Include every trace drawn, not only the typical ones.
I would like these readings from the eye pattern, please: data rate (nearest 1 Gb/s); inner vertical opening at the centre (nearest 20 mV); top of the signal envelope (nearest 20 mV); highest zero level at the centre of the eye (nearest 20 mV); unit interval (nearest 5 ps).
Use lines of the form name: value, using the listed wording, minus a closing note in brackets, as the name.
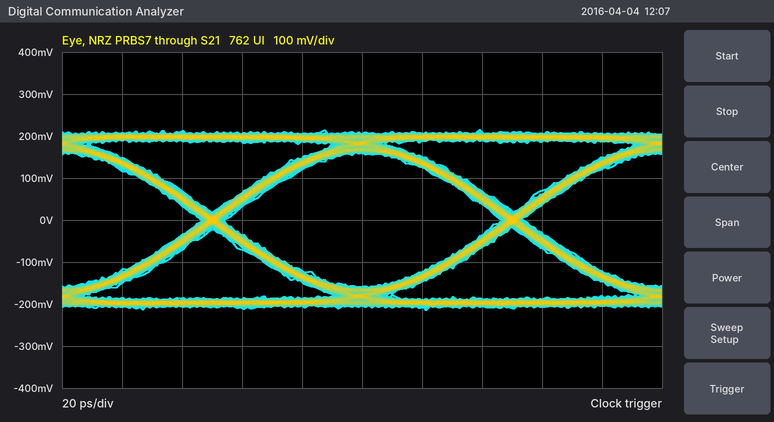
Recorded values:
data rate: 10 Gb/s
inner vertical opening at the centre: 320 mV
top of the signal envelope: 220 mV
highest zero level at the centre of the eye: -160 mV
unit interval: 100 ps
